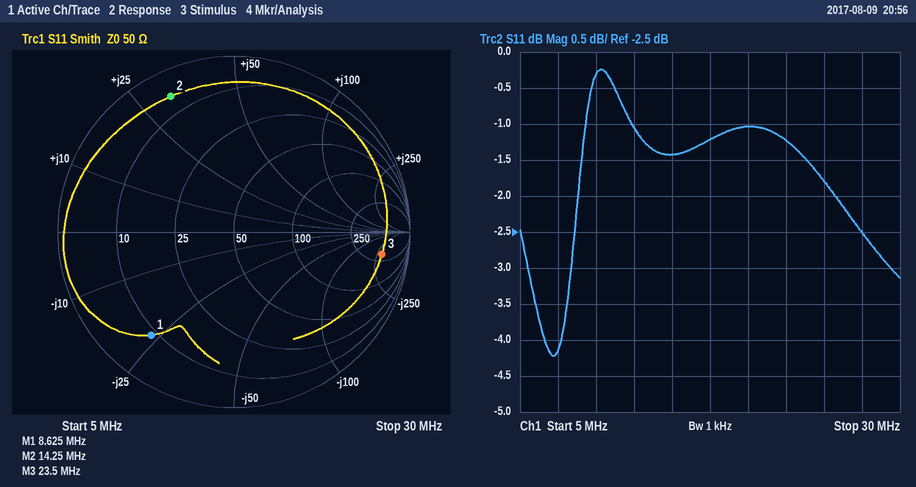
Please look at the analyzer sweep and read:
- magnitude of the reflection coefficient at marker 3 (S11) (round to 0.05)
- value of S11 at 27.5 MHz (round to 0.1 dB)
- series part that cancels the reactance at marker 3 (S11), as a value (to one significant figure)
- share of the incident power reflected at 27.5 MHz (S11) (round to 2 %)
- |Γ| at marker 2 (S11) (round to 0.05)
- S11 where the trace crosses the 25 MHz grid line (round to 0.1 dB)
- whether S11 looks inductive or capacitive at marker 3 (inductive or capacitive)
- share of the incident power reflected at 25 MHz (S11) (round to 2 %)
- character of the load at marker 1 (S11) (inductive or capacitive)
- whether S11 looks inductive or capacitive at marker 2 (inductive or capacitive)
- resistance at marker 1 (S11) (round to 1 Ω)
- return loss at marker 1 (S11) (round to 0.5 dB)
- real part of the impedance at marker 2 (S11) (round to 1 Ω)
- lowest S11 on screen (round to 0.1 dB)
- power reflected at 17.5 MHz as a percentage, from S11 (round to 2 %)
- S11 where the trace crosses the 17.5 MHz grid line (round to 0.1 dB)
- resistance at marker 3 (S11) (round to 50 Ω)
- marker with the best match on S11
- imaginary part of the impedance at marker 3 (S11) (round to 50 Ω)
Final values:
0.85
-2.5 dB
2 µH
56 %
0.85
-1.8 dB
capacitive
66 %
capacitive
inductive
9 Ω
2.5 dB
6 Ω
-4.2 dB
76 %
-1.2 dB
350 Ω
marker 1
-300 Ω
